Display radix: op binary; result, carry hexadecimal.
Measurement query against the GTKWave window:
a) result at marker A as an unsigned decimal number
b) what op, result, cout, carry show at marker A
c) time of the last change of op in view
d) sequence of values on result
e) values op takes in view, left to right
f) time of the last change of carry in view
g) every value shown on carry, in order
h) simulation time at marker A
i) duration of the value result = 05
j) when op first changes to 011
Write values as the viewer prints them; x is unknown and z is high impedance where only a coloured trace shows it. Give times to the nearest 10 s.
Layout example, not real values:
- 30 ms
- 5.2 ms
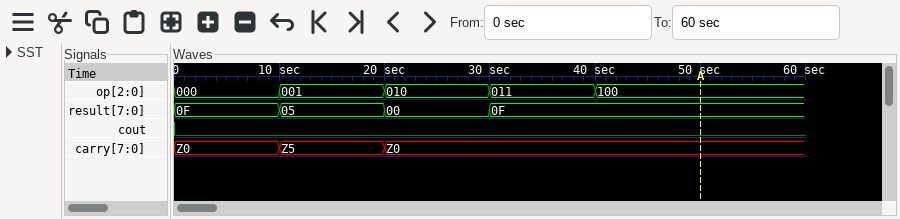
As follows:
- 15
- op=100, result=0F, cout=0, carry=Z0
- 40 s
- 0F, 05, 00, 0F
- 000, 001, 010, 011, 100
- 20 s
- Z0, Z5, Z0
- 50 s
- 10 s
- 30 s
